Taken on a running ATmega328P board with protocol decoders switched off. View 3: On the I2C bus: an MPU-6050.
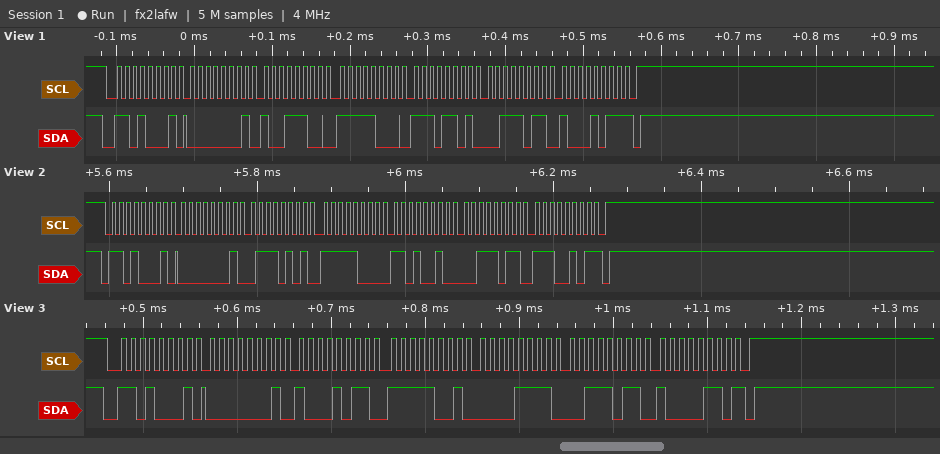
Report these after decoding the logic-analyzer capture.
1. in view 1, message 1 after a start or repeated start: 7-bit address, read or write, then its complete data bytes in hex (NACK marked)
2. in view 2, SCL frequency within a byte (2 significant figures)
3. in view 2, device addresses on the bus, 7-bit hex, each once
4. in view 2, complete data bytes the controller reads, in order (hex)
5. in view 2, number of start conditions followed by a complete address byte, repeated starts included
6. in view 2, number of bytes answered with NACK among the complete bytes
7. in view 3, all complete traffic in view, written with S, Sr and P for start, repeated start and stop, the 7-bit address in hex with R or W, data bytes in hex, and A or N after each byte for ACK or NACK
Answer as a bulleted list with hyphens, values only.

- 0x68 read: 01 9C F8 ED 3B 8B NACK
- 100 kHz
- 0x68
- 01 75 F8 D2 3B E5
- 1
- 1
- S 68R A 01 A 8B A F9 A 0F A 3B A 86 N P
